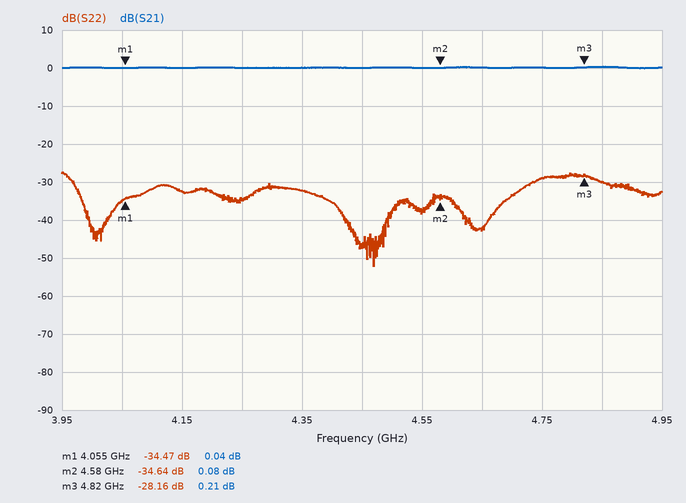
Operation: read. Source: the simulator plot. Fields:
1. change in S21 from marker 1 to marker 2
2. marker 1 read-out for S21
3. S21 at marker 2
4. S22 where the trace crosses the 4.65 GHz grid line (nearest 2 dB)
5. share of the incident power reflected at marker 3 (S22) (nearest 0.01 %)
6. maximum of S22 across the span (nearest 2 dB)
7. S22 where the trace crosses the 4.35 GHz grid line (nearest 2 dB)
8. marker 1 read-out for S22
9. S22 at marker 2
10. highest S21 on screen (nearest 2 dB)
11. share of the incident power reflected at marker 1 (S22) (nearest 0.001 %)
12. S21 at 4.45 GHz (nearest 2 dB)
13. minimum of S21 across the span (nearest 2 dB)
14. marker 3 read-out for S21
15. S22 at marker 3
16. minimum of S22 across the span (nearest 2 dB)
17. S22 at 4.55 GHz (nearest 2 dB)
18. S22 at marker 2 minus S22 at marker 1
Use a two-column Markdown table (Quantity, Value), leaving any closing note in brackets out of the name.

| Quantity | Value |
|---|---|
| change in S21 from marker 1 to marker 2 | 0.04 dB |
| marker 1 read-out for S21 | 0.04 dB |
| S21 at marker 2 | 0.08 dB |
| S22 where the trace crosses the 4.65 GHz grid line | -42 dB |
| share of the incident power reflected at marker 3 (S22) | 0.15 % |
| maximum of S22 across the span | -28 dB |
| S22 where the trace crosses the 4.35 GHz grid line | -32 dB |
| marker 1 read-out for S22 | -34.47 dB |
| S22 at marker 2 | -34.64 dB |
| highest S21 on screen | 0 dB |
| share of the incident power reflected at marker 1 (S22) | 0.036 % |
| S21 at 4.45 GHz | 0 dB |
| minimum of S21 across the span | 0 dB |
| marker 3 read-out for S21 | 0.21 dB |
| S22 at marker 3 | -28.16 dB |
| minimum of S22 across the span | -52 dB |
| S22 at 4.55 GHz | -38 dB |
| S22 at marker 2 minus S22 at marker 1 | -0.17 dB |
